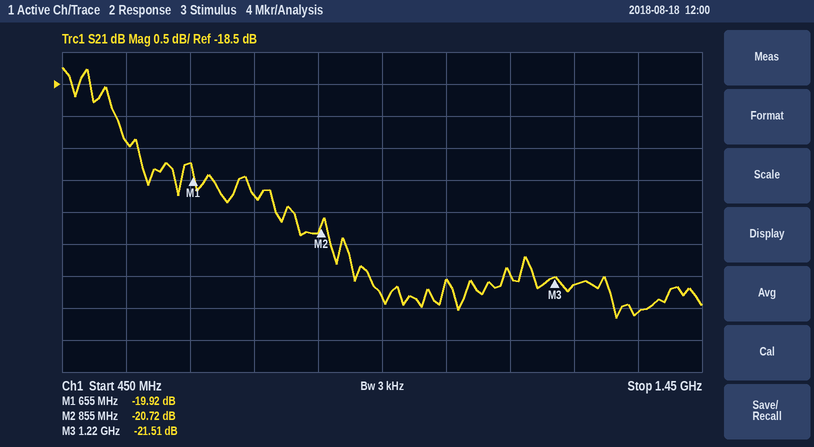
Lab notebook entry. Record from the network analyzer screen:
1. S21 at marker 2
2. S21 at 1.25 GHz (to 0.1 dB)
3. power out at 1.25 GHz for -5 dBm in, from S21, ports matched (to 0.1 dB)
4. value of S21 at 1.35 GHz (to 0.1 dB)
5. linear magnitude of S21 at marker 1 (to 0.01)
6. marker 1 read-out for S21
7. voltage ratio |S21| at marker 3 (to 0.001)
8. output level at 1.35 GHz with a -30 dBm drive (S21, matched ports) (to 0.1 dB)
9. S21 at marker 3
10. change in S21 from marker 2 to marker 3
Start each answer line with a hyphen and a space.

- -20.72 dB
- -21.6 dB
- -26.6 dBm
- -22.1 dB
- 0.10
- -19.92 dB
- 0.084
- -52.1 dBm
- -21.51 dB
- -0.79 dB
